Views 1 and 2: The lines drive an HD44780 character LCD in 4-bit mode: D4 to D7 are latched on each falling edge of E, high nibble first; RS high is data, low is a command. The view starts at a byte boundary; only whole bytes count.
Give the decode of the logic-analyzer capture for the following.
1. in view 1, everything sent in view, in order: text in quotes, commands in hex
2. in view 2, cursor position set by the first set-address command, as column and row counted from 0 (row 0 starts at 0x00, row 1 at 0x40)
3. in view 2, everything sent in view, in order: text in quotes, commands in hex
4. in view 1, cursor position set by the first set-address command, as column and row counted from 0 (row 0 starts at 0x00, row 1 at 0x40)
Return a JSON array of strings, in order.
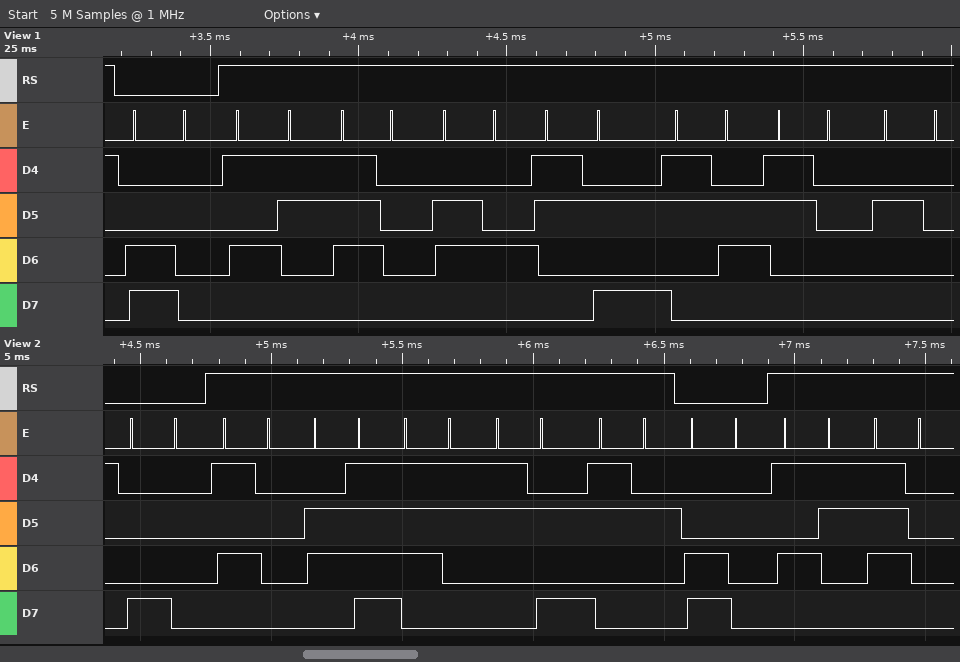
["0xC0 \"Spd:60 \"", "column 0, row 0", "0x80 \"Pos:2\" 0xC0 \"Sp\"", "column 0, row 1"]
